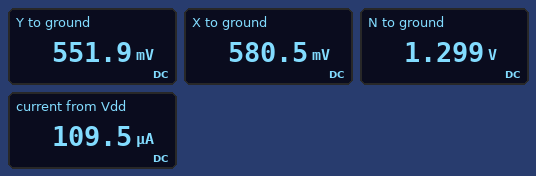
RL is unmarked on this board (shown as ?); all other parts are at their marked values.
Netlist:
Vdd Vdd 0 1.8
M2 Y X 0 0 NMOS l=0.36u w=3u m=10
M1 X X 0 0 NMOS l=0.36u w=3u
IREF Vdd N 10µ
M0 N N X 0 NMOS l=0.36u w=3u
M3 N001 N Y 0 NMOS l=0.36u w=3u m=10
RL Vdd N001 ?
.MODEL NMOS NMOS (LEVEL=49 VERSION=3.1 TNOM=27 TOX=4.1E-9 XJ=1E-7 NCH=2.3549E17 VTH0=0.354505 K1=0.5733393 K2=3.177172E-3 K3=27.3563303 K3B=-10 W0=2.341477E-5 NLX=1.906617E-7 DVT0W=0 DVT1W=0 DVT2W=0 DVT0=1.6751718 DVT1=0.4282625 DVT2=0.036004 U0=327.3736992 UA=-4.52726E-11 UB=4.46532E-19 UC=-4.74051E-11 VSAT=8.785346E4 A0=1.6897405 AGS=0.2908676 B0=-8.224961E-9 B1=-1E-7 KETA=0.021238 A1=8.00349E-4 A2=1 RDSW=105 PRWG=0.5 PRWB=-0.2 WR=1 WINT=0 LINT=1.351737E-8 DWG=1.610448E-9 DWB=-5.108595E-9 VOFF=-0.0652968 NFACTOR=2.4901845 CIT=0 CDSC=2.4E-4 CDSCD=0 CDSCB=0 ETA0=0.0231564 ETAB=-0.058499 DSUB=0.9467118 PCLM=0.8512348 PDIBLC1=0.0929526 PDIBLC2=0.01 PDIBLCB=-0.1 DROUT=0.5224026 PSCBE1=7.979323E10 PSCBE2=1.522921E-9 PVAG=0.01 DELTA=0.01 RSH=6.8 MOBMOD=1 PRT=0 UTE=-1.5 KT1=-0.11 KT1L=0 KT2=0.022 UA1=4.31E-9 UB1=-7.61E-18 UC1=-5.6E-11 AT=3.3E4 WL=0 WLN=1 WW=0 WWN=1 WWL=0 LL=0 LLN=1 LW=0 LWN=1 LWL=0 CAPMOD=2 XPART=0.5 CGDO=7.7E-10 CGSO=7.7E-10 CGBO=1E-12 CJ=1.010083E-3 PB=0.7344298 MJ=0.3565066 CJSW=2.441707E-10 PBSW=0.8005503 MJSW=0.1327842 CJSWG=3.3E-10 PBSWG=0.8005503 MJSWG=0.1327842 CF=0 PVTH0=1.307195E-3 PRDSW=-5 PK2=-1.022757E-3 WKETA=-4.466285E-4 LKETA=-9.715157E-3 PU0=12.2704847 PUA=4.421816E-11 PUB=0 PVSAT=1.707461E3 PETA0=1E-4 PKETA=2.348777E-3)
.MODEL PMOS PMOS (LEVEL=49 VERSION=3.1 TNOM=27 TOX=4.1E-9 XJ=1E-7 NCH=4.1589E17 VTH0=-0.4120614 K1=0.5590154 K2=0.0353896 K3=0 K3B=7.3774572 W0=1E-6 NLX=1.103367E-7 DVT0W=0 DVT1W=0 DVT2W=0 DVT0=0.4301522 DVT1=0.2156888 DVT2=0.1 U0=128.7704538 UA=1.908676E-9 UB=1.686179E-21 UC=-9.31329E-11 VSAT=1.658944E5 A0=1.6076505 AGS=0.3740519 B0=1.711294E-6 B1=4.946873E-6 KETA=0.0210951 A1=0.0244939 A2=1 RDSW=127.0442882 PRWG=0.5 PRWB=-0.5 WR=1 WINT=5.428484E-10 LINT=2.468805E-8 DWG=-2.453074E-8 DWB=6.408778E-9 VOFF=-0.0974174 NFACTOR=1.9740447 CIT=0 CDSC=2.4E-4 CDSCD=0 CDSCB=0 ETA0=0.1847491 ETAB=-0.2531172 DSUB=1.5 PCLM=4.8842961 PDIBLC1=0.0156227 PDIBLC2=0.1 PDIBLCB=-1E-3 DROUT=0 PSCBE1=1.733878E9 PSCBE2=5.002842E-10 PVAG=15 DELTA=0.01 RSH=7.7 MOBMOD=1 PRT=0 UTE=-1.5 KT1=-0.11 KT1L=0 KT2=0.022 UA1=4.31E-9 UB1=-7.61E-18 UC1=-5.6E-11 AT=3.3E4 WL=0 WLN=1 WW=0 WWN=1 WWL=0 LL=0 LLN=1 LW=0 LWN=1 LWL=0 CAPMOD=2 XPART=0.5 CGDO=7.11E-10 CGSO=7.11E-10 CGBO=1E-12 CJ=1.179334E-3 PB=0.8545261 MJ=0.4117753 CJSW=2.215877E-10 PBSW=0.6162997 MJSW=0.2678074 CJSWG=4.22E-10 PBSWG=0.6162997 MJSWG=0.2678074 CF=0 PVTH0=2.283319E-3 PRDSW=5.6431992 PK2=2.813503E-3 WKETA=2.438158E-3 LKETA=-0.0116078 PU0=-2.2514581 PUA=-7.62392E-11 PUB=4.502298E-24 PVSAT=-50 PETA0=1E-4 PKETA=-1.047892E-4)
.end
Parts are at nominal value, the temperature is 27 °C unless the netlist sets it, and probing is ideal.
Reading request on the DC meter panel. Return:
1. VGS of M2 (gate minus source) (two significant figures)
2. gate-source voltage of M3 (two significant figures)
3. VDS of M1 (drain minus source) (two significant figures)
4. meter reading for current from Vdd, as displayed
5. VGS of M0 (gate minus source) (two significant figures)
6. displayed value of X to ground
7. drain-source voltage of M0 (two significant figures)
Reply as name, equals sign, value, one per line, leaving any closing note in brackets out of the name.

VGS of M2 (gate minus source) = 580 mV
gate-source voltage of M3 = 750 mV
VDS of M1 (drain minus source) = 580 mV
meter reading for current from Vdd, as displayed = 109.5 µA
VGS of M0 (gate minus source) = 720 mV
displayed value of X to ground = 580.5 mV
drain-source voltage of M0 = 720 mV
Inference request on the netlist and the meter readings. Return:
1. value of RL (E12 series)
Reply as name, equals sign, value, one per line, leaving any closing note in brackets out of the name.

value of RL = 12 kΩ
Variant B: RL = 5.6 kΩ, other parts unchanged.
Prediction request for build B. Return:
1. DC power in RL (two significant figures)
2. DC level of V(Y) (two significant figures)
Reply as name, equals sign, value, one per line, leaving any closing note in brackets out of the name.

DC power in RL = 56 µW
DC level of V(Y) = 580 mV
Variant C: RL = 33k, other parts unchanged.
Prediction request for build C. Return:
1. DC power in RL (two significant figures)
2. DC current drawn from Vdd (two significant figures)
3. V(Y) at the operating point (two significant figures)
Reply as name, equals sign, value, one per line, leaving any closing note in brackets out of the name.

DC power in RL = 94 µW
DC current drawn from Vdd = 63 µA
V(Y) at the operating point = 39 mV
